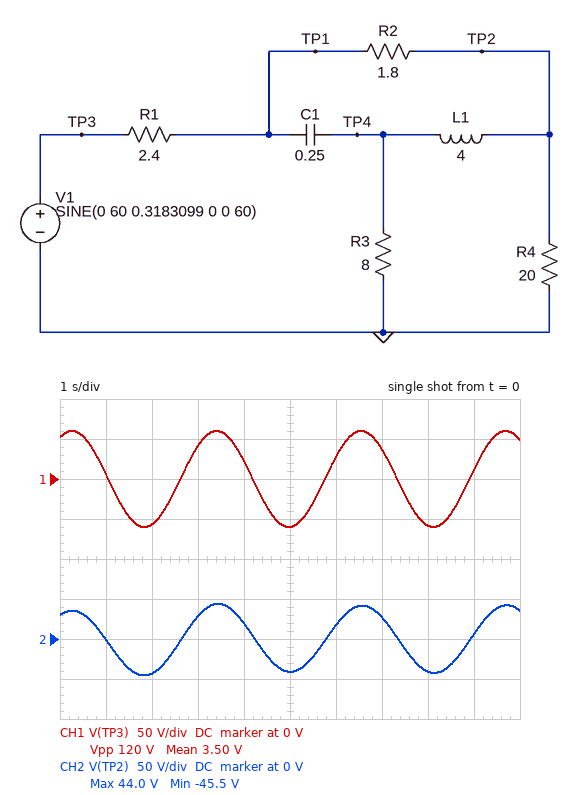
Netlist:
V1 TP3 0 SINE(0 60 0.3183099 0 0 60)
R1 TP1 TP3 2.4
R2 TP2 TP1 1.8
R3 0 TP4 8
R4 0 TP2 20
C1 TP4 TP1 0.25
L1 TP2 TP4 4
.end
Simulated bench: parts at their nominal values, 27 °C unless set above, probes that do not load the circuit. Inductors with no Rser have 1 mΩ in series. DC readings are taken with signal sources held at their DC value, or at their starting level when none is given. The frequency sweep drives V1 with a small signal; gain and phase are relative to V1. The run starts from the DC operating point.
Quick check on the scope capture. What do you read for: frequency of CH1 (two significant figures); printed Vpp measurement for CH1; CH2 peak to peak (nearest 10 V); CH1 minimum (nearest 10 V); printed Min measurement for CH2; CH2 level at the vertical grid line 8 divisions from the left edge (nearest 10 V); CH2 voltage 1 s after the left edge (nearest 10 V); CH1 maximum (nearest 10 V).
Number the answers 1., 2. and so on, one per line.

1. 320 mHz
2. 120 V
3. 90 V
4. -60 V
5. -45.5 V
6. -40 V
7. 0 V
8. 60 V
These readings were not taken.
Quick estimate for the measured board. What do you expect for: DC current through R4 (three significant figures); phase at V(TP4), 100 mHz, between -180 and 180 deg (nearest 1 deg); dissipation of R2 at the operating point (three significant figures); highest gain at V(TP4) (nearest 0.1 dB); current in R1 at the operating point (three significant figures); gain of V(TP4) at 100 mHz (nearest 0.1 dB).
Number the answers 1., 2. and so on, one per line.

1. 1.50 A
2. -8 deg
3. 49.4 W
4. -3.0 dB
5. 5.24 A
6. -6.7 dB
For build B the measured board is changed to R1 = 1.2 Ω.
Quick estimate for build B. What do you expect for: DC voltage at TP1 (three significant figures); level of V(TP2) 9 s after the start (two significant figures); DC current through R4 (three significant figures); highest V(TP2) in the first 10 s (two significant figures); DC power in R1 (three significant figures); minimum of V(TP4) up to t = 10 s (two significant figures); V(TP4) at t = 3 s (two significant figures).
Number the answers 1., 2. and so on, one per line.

1. 44.8 V
2. 8.5 V
3. 1.70 A
4. 51 V
5. 42.7 W
6. -51 V
7. 46 V
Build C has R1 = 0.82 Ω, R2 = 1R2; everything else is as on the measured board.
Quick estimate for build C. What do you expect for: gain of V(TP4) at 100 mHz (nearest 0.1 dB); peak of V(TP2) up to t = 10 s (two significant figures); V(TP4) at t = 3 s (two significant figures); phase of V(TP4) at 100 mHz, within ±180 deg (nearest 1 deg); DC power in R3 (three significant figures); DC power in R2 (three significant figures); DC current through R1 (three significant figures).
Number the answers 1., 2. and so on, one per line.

1. -4.6 dB
2. 54 V
3. 49 V
4. -15 deg
5. 184 W
6. 54.2 W
7. 6.72 A
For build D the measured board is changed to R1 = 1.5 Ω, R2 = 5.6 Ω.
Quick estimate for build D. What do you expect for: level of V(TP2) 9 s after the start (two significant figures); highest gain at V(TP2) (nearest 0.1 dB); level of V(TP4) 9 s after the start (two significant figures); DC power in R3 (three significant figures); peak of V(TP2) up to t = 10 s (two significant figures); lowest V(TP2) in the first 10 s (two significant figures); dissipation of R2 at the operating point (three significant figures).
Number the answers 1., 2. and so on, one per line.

1. 7.4 V
2. -1.9 dB
3. 21 V
4. 67.1 W
5. 46 V
6. -51 V
7. 92.1 W
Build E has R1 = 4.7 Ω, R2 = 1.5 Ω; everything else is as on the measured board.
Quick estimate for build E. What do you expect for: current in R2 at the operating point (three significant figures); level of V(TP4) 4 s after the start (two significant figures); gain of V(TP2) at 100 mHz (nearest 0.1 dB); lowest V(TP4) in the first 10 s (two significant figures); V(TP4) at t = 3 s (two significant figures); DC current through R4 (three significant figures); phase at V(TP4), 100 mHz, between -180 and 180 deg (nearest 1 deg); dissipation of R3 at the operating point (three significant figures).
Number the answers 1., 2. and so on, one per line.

1. 4.36 A
2. 4.2 V
3. -5.6 dB
4. -35 V
5. 30 V
6. 1.25 A
7. -10 deg
8. 77.6 W
